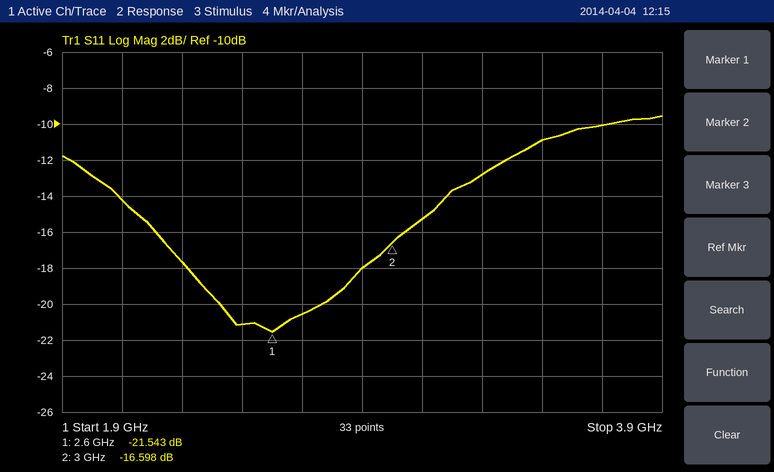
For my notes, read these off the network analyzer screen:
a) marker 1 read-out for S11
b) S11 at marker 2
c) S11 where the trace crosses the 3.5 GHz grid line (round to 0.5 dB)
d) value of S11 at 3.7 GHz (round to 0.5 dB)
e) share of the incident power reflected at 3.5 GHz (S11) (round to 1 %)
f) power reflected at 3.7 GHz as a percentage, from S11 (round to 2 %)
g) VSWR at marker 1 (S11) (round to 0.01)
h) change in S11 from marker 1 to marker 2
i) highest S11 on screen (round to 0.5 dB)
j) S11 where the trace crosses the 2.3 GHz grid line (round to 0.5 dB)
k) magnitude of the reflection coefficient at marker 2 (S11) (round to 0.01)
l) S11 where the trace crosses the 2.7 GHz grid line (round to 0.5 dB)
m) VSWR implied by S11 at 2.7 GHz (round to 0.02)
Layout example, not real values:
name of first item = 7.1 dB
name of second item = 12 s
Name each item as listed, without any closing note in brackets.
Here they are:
marker 1 read-out for S11 = -21.543 dB
S11 at marker 2 = -16.598 dB
S11 where the trace crosses the 3.5 GHz grid line = -11.0 dB
value of S11 at 3.7 GHz = -10.0 dB
share of the incident power reflected at 3.5 GHz (S11) = 8 %
power reflected at 3.7 GHz as a percentage, from S11 = 10 %
VSWR at marker 1 (S11) = 1.18
change in S11 from marker 1 to marker 2 = 4.945 dB
highest S11 on screen = -9.5 dB
S11 where the trace crosses the 2.3 GHz grid line = -17.5 dB
magnitude of the reflection coefficient at marker 2 (S11) = 0.15
S11 where the trace crosses the 2.7 GHz grid line = -20.5 dB
VSWR implied by S11 at 2.7 GHz = 1.20
